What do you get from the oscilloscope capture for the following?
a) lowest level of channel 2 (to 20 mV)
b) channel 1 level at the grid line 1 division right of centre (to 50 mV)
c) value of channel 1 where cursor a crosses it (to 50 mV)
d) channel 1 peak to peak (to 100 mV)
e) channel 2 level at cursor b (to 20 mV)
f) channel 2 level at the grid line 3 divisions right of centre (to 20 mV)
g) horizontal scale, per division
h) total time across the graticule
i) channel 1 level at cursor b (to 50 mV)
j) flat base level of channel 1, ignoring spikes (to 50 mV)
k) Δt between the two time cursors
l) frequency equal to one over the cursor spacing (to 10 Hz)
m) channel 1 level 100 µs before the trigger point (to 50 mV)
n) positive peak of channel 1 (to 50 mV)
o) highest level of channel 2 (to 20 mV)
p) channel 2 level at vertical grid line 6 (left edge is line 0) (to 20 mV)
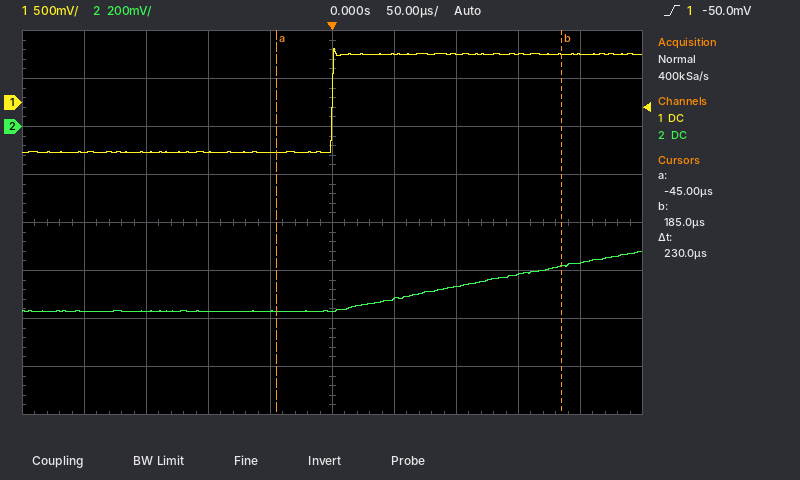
-780 mV
500 mV
-500 mV
1.10 V
-580 mV
-620 mV
50 µs
500 µs
500 mV
-500 mV
230 µs
4.35 kHz
-500 mV
550 mV
-520 mV
-720 mV
